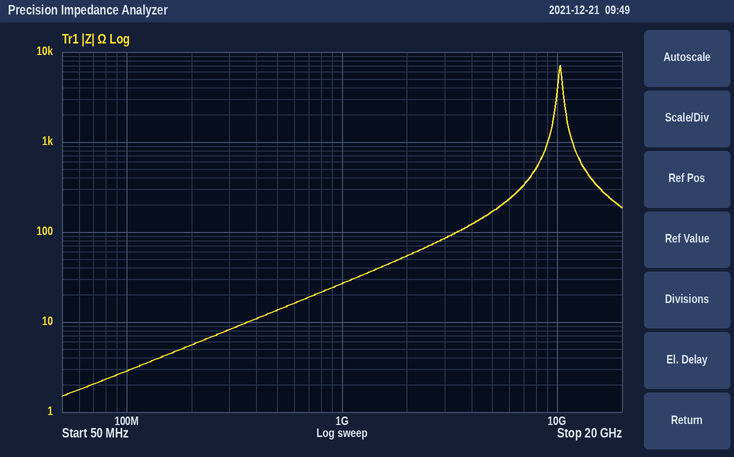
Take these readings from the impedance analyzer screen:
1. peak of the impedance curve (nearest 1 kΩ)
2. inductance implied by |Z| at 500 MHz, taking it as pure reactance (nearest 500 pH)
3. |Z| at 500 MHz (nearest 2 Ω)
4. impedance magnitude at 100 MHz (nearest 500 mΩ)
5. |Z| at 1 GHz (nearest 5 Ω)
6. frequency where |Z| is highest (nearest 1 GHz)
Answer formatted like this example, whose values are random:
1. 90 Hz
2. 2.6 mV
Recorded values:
1. 7 kΩ
2. 4.5 nH
3. 14 Ω
4. 3.0 Ω
5. 25 Ω
6. 10 GHz
